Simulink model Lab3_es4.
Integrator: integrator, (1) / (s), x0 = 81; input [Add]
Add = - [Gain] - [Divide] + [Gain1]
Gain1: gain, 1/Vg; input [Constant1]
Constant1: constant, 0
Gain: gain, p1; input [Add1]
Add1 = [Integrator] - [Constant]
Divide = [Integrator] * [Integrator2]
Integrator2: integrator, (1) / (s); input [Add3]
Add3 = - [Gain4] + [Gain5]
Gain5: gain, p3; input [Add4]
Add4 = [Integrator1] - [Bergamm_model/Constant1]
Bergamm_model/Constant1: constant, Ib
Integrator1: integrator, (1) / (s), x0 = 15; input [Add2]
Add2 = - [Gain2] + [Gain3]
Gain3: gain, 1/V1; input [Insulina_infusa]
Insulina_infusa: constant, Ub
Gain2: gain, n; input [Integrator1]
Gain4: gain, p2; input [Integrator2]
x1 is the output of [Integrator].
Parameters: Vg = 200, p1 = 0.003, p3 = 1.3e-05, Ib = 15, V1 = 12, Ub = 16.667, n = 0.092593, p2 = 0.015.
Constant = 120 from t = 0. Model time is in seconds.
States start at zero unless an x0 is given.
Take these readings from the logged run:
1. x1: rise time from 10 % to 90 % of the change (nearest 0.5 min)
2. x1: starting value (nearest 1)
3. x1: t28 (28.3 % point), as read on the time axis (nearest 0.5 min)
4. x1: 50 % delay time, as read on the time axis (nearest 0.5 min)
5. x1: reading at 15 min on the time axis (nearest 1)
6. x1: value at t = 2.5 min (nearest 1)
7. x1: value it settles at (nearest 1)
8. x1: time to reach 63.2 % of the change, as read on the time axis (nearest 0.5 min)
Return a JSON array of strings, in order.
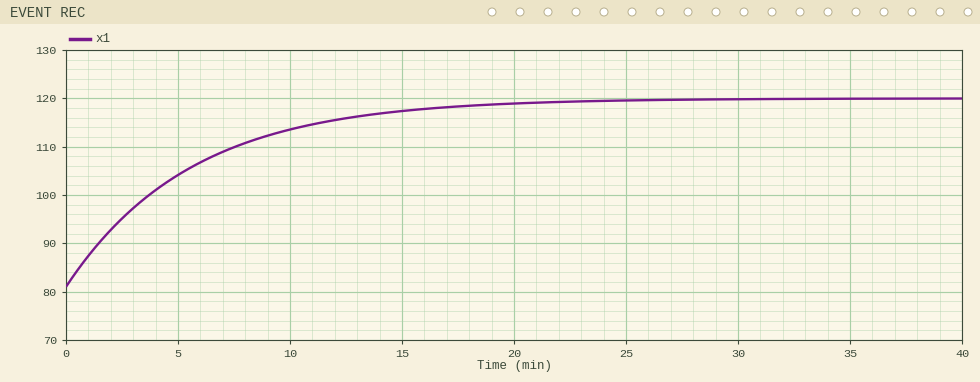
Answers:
["12.0 min", "81", "2.0 min", "4.0 min", "117", "95", "120", "5.5 min"]
